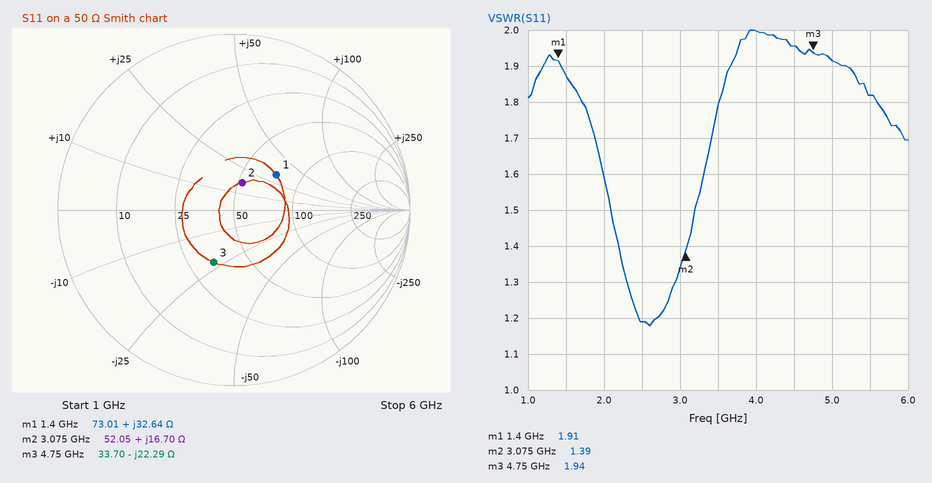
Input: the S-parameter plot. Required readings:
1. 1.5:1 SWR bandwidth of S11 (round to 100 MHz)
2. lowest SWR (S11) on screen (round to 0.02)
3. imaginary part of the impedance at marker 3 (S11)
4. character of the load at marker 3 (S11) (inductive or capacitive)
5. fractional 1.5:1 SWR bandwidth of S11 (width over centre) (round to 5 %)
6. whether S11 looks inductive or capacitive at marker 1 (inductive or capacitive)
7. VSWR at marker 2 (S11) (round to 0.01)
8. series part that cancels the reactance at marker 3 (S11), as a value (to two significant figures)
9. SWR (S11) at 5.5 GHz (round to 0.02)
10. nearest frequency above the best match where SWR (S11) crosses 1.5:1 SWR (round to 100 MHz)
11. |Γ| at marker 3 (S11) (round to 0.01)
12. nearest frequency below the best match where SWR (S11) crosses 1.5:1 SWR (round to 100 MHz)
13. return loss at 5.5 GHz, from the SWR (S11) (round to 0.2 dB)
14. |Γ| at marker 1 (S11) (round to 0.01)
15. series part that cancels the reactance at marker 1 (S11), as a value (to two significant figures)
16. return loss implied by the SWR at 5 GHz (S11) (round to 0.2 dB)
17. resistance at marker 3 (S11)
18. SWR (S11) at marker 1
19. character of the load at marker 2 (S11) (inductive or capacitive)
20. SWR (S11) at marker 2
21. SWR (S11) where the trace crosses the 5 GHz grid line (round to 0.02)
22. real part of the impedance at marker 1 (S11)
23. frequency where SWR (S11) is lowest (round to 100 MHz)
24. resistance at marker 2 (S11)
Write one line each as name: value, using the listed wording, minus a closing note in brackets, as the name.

1.5:1 SWR bandwidth of S11: 1.1 GHz
lowest SWR (S11) on screen: 1.18
imaginary part of the impedance at marker 3: -22.29 Ω
character of the load at marker 3 (S11): capacitive
fractional 1.5:1 SWR bandwidth of S11 (width over centre): 40 %
whether S11 looks inductive or capacitive at marker 1: inductive
VSWR at marker 2 (S11): 1.39
series part that cancels the reactance at marker 3 (S11), as a value: 750 pH
SWR (S11) at 5.5 GHz: 1.82
nearest frequency above the best match where SWR (S11) crosses 1.5:1 SWR: 3.2 GHz
|Γ| at marker 3 (S11): 0.32
nearest frequency below the best match where SWR (S11) crosses 1.5:1 SWR: 2.1 GHz
return loss at 5.5 GHz, from the SWR (S11): 10.8 dB
|Γ| at marker 1 (S11): 0.31
series part that cancels the reactance at marker 1 (S11), as a value: 3.5 pF
return loss implied by the SWR at 5 GHz (S11): 10.0 dB
resistance at marker 3: 33.70 Ω
SWR (S11) at marker 1: 1.91
character of the load at marker 2 (S11): inductive
SWR (S11) at marker 2: 1.39
SWR (S11) where the trace crosses the 5 GHz grid line: 1.92
real part of the impedance at marker 1: 73.01 Ω
frequency where SWR (S11) is lowest: 2.6 GHz
resistance at marker 2: 52.05 Ω
